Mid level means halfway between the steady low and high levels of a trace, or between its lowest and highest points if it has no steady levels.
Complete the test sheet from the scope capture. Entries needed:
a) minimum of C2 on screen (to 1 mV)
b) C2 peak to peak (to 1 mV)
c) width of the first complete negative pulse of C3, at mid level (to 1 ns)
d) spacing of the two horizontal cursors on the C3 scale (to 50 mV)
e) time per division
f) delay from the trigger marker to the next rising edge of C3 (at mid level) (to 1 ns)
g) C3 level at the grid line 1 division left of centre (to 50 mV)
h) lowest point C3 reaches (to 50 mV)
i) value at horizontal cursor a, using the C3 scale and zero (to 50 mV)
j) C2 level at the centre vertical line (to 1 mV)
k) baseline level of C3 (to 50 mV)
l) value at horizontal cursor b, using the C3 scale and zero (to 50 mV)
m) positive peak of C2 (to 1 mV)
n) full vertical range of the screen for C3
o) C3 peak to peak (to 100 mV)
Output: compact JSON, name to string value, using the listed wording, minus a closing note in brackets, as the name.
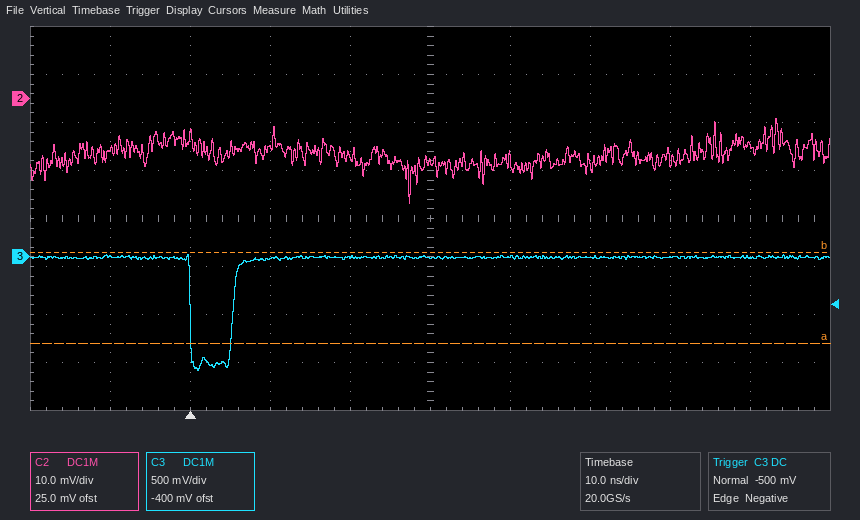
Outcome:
{"minimum of C2 on screen": "-22 mV", "C2 peak to peak": "18 mV", "width of the first complete negative pulse of C3, at mid level": "5 ns", "spacing of the two horizontal cursors on the C3 scale": "950 mV", "time per division": "10 ns", "delay from the trigger marker to the next rising edge of C3 (at mid level)": "5 ns", "C3 level at the grid line 1 division left of centre": "0 mV", "lowest point C3 reaches": "-1.20 V", "value at horizontal cursor a, using the C3 scale and zero": "-900 mV", "C2 level at the centre vertical line": "-13 mV", "baseline level of C3": "0 mV", "value at horizontal cursor b, using the C3 scale and zero": "50 mV", "positive peak of C2": "-4 mV", "full vertical range of the screen for C3": "4 V", "C3 peak to peak": "1.20 V"}
